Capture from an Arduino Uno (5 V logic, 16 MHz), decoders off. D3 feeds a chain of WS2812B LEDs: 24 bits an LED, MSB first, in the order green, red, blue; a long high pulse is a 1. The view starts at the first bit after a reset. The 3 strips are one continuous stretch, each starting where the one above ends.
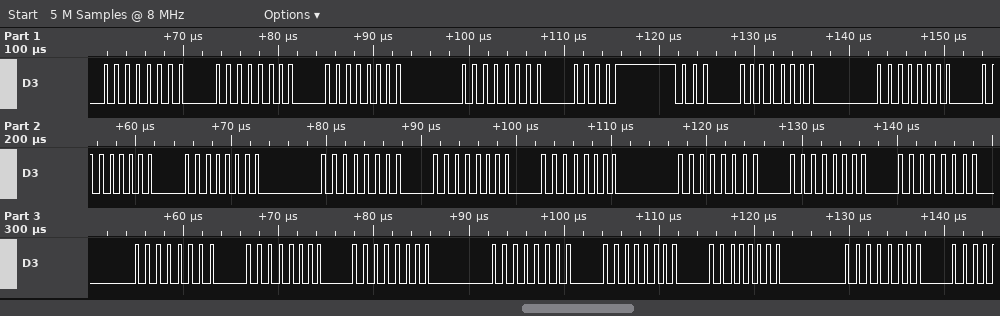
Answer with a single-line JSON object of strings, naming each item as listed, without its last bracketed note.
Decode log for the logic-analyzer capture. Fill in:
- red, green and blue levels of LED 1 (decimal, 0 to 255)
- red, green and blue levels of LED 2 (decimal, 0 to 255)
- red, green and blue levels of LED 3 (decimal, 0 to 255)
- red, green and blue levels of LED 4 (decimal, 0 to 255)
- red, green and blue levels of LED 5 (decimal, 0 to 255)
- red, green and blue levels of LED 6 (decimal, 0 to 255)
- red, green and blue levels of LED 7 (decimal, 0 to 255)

{"red, green and blue levels of LED 1": "0, 0, 0", "red, green and blue levels of LED 2": "8, 0, 0", "red, green and blue levels of LED 3": "0, 0, 0", "red, green and blue levels of LED 4": "0, 0, 0", "red, green and blue levels of LED 5": "0, 0, 0", "red, green and blue levels of LED 6": "0, 0, 0", "red, green and blue levels of LED 7": "0, 0, 0"}
